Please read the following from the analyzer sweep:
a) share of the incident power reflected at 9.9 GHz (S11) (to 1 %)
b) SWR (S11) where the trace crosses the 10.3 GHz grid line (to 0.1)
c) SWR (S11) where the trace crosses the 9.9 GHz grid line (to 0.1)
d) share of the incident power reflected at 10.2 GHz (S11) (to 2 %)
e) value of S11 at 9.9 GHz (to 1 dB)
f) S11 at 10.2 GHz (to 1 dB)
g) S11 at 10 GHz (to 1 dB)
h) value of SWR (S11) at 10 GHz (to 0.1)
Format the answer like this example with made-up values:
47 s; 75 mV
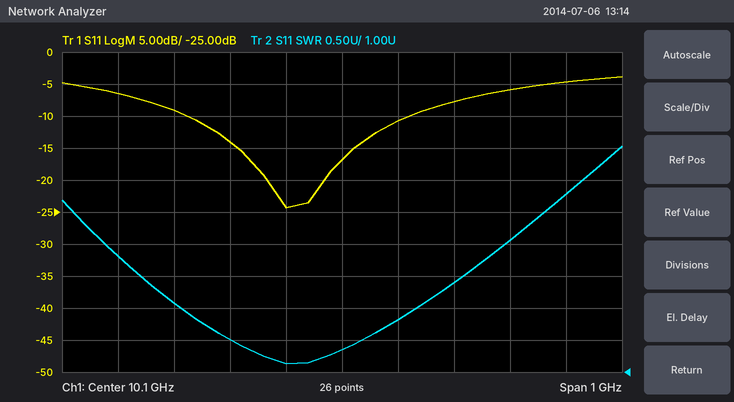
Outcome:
4 %; 2.4; 1.5; 8 %; -14 dB; -11 dB; -24 dB; 1.1
